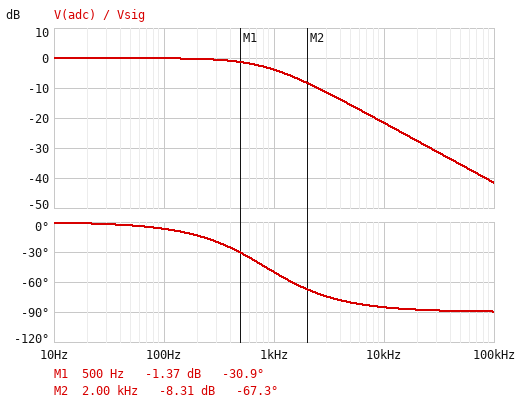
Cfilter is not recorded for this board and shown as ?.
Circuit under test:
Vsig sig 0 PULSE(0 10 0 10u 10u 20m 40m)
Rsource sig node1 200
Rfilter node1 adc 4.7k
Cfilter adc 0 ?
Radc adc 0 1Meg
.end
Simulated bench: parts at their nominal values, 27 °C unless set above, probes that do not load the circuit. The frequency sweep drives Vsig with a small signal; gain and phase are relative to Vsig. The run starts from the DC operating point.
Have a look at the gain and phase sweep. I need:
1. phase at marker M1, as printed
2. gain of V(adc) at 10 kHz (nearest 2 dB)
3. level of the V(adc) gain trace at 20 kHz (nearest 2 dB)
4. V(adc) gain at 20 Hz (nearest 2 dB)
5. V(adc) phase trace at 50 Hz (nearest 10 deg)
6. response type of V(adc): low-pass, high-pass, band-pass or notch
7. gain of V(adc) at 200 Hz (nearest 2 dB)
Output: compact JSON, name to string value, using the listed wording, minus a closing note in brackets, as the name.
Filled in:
{"phase at marker M1, as printed": "-30.9 deg", "gain of V(adc) at 10 kHz": "-22 dB", "level of the V(adc) gain trace at 20 kHz": "-28 dB", "V(adc) gain at 20 Hz": "0 dB", "V(adc) phase trace at 50 Hz": "0 deg", "response type of V(adc): low-pass, high-pass, band-pass or notch": "low-pass", "gain of V(adc) at 200 Hz": "0 dB"}
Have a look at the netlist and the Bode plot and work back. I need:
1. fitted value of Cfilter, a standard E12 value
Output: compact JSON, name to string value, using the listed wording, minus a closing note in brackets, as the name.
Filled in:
{"fitted value of Cfilter, a standard E12 value": "39 nF"}
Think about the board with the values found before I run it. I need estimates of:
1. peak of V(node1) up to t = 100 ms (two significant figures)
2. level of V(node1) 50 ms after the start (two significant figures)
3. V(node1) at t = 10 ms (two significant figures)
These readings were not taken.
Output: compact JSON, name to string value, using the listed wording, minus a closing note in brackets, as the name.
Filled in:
{"peak of V(node1) up to t = 100 ms": "10 V", "level of V(node1) 50 ms after the start": "10 V", "V(node1) at t = 10 ms": "10 V"}
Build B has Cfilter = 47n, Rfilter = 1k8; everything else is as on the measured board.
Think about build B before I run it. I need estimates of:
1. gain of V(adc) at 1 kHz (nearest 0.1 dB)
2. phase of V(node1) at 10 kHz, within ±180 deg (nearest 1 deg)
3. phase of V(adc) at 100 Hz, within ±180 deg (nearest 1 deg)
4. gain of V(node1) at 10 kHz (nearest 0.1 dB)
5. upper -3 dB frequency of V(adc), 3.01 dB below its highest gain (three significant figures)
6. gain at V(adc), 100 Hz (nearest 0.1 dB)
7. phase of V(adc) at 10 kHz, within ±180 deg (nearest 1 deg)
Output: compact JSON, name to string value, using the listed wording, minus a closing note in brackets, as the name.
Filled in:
{"gain of V(adc) at 1 kHz": "-1.3 dB", "phase of V(node1) at 10 kHz, within ±180 deg": "-1 deg", "phase of V(adc) at 100 Hz, within ±180 deg": "-3 deg", "gain of V(node1) at 10 kHz": "-0.9 dB", "upper -3 dB frequency of V(adc), 3.01 dB below its highest gain": "1.70 kHz", "gain at V(adc), 100 Hz": "0 dB", "phase of V(adc) at 10 kHz, within ±180 deg": "-80 deg"}
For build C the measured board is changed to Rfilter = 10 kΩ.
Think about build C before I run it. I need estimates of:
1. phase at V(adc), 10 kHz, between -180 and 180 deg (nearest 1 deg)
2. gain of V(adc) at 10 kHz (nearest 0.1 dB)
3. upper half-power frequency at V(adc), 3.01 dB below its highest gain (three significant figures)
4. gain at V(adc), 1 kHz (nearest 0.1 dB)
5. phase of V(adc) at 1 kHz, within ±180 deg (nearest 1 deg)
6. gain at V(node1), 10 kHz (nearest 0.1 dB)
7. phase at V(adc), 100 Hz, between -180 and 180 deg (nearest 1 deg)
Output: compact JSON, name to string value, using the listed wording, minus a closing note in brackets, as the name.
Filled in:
{"phase at V(adc), 10 kHz, between -180 and 180 deg": "-88 deg", "gain of V(adc) at 10 kHz": "-28.0 dB", "upper half-power frequency at V(adc), 3.01 dB below its highest gain": "404 Hz", "gain at V(adc), 1 kHz": "-8.6 dB", "phase of V(adc) at 1 kHz, within ±180 deg": "-68 deg", "gain at V(node1), 10 kHz": "-0.2 dB", "phase at V(adc), 100 Hz, between -180 and 180 deg": "-14 deg"}
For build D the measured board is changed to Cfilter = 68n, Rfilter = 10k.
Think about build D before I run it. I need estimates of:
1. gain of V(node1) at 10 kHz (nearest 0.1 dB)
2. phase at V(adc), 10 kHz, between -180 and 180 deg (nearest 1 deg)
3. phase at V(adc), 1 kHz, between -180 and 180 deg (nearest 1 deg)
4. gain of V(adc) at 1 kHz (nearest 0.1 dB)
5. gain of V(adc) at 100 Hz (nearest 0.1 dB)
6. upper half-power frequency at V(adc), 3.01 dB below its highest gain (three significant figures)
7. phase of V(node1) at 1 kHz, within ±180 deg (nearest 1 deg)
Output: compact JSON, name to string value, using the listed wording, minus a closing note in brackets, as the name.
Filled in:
{"gain of V(node1) at 10 kHz": "-0.2 dB", "phase at V(adc), 10 kHz, between -180 and 180 deg": "-89 deg", "phase at V(adc), 1 kHz, between -180 and 180 deg": "-77 deg", "gain of V(adc) at 1 kHz": "-13.0 dB", "gain of V(adc) at 100 Hz": "-0.8 dB", "upper half-power frequency at V(adc), 3.01 dB below its highest gain": "232 Hz", "phase of V(node1) at 1 kHz, within ±180 deg": "0 deg"}
